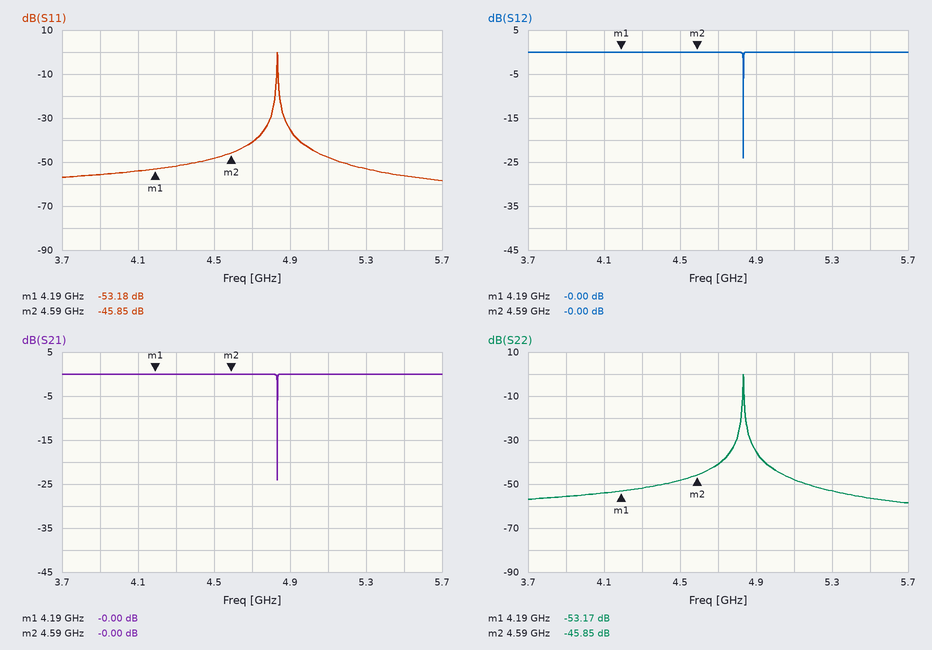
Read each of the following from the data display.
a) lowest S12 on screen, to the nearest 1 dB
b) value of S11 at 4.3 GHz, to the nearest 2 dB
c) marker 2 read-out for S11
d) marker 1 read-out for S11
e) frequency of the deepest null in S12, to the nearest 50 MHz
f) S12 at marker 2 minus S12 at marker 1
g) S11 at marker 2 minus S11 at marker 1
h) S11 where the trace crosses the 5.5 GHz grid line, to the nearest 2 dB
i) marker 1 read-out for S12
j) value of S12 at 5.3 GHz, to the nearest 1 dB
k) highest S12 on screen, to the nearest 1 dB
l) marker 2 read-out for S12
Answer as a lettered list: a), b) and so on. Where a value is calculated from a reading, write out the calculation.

a) -24 dB
b) -52 dB
c) -45.85 dB
d) -53.18 dB
e) 4.85 GHz
f) -0 − (-0) = 0.00 dB
g) -45.85 − (-53.18) = 7.33 dB
h) -56 dB
i) -0.00 dB
j) 0 dB
k) 0 dB
l) -0.00 dB
